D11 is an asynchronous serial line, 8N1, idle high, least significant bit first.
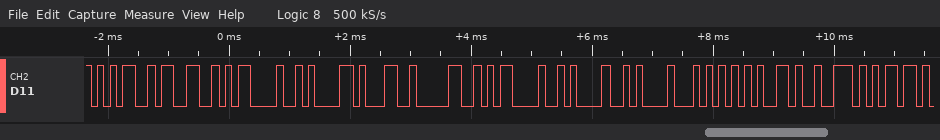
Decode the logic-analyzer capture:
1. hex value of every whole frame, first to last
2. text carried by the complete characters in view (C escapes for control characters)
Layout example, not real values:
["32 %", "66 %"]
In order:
["35 33 0D 0A 31 30 0D 0A 0A 54 65 72 6D", "\"53\\r\\n10\\r\\n\\nTerm\""]
